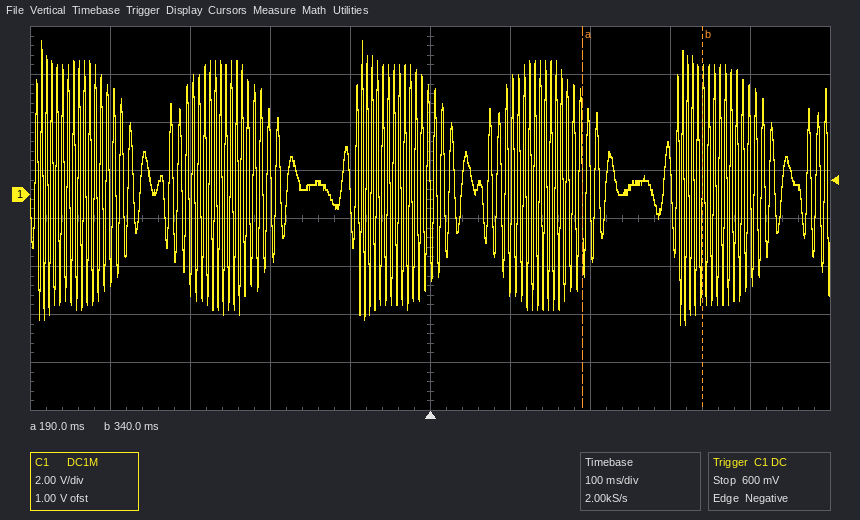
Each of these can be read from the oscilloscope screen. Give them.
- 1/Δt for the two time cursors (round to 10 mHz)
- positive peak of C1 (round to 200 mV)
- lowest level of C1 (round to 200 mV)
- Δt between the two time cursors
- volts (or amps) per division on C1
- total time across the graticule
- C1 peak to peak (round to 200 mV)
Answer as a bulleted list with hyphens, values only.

- 6.67 Hz
- 6.4 V
- -5.4 V
- 150 ms
- 2 V
- 1 s
- 11.8 V
